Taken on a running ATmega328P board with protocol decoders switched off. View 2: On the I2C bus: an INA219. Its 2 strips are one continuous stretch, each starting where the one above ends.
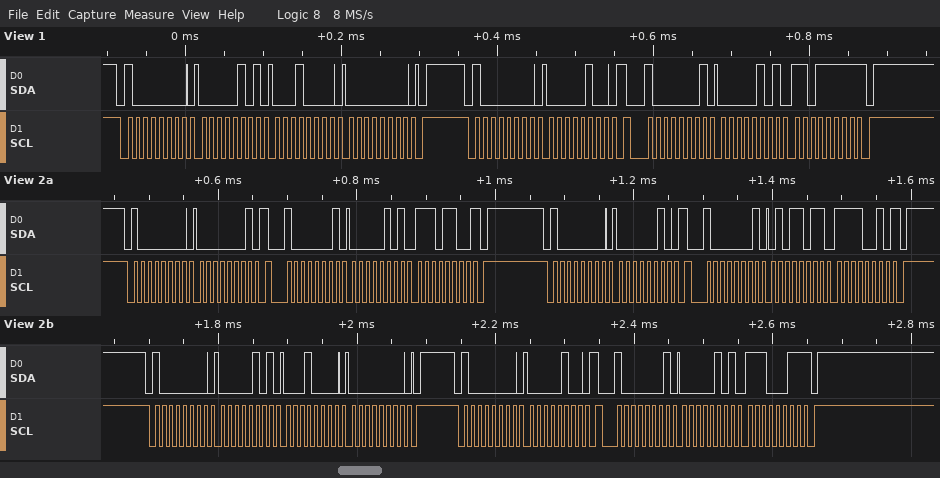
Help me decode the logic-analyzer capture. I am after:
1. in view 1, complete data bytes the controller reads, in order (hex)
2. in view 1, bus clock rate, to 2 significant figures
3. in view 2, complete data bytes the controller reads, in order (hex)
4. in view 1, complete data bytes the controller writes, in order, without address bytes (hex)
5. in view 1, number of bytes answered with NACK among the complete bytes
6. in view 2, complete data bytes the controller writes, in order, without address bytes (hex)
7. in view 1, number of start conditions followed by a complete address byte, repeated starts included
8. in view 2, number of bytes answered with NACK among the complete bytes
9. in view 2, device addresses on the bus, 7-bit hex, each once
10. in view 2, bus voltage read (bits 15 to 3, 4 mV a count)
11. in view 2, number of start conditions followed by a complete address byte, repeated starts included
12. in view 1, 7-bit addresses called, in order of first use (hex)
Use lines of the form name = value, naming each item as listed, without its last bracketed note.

in view 1, complete data bytes the controller reads, in order = 05 DF
in view 1, bus clock rate, to 2 significant figures = 100 kHz
in view 2, complete data bytes the controller reads, in order = 05 EC 5B F2 05 E3
in view 1, complete data bytes the controller writes, in order, without address bytes = 05 10 00 04
in view 1, number of bytes answered with NACK among the complete bytes = 1
in view 2, complete data bytes the controller writes, in order, without address bytes = 01 02 05 10 00 04
in view 1, number of start conditions followed by a complete address byte, repeated starts included = 3
in view 2, number of bytes answered with NACK among the complete bytes = 3
in view 2, device addresses on the bus, 7-bit hex, each once = 0x40
in view 2, bus voltage read = 11.768 V
in view 2, number of start conditions followed by a complete address byte, repeated starts included = 7
in view 1, 7-bit addresses called, in order of first use = 0x40
